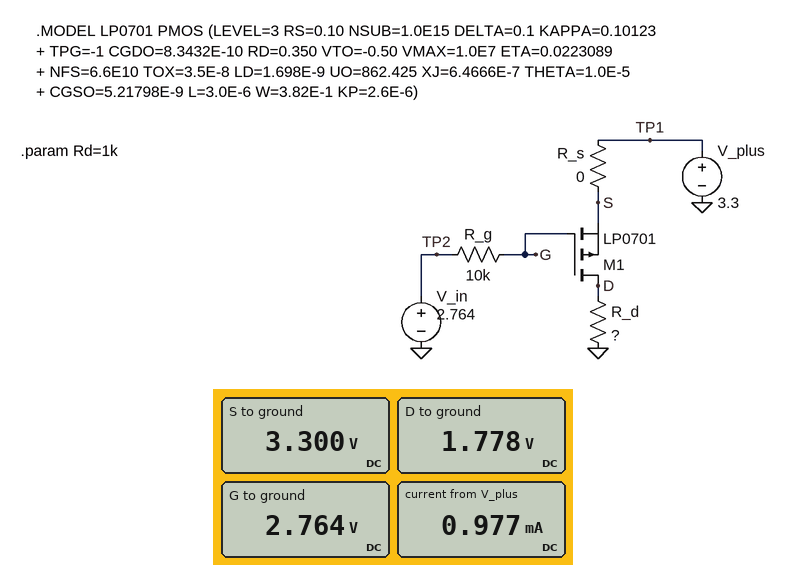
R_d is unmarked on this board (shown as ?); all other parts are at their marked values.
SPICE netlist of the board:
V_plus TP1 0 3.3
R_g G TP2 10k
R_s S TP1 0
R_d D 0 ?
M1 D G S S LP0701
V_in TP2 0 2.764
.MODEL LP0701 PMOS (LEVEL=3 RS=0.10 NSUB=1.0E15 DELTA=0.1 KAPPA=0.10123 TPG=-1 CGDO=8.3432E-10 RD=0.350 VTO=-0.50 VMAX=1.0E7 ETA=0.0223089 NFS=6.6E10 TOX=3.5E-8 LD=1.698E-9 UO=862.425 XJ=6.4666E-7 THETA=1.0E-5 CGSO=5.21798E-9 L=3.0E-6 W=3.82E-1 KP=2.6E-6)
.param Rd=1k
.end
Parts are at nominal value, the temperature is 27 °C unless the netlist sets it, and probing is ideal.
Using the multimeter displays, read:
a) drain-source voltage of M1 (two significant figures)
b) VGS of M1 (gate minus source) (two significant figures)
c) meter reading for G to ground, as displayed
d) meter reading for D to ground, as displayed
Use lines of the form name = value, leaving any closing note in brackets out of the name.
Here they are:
drain-source voltage of M1 = -1.5 V
VGS of M1 (gate minus source) = -540 mV
meter reading for G to ground, as displayed = 2.764 V
meter reading for D to ground, as displayed = 1.778 V
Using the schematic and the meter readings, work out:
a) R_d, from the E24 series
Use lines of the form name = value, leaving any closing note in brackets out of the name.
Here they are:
R_d, from the E24 series = 2.7 kΩ
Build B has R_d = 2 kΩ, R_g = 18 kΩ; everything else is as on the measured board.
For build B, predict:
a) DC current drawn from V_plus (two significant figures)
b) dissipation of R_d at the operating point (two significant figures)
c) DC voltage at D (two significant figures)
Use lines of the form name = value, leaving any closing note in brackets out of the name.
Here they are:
DC current drawn from V_plus = 490 µA
dissipation of R_d at the operating point = 880 µW
DC voltage at D = 1.3 V
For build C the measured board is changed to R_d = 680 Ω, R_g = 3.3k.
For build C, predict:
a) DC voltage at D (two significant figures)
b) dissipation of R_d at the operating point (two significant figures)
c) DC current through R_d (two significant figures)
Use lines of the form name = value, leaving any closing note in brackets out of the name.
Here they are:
DC voltage at D = 460 mV
dissipation of R_d at the operating point = 310 µW
DC current through R_d = 680 µA
